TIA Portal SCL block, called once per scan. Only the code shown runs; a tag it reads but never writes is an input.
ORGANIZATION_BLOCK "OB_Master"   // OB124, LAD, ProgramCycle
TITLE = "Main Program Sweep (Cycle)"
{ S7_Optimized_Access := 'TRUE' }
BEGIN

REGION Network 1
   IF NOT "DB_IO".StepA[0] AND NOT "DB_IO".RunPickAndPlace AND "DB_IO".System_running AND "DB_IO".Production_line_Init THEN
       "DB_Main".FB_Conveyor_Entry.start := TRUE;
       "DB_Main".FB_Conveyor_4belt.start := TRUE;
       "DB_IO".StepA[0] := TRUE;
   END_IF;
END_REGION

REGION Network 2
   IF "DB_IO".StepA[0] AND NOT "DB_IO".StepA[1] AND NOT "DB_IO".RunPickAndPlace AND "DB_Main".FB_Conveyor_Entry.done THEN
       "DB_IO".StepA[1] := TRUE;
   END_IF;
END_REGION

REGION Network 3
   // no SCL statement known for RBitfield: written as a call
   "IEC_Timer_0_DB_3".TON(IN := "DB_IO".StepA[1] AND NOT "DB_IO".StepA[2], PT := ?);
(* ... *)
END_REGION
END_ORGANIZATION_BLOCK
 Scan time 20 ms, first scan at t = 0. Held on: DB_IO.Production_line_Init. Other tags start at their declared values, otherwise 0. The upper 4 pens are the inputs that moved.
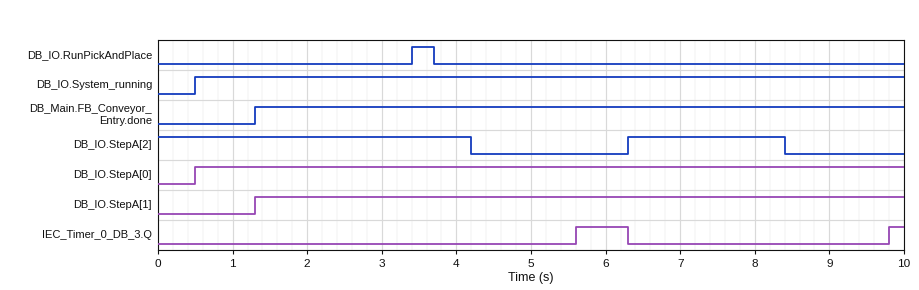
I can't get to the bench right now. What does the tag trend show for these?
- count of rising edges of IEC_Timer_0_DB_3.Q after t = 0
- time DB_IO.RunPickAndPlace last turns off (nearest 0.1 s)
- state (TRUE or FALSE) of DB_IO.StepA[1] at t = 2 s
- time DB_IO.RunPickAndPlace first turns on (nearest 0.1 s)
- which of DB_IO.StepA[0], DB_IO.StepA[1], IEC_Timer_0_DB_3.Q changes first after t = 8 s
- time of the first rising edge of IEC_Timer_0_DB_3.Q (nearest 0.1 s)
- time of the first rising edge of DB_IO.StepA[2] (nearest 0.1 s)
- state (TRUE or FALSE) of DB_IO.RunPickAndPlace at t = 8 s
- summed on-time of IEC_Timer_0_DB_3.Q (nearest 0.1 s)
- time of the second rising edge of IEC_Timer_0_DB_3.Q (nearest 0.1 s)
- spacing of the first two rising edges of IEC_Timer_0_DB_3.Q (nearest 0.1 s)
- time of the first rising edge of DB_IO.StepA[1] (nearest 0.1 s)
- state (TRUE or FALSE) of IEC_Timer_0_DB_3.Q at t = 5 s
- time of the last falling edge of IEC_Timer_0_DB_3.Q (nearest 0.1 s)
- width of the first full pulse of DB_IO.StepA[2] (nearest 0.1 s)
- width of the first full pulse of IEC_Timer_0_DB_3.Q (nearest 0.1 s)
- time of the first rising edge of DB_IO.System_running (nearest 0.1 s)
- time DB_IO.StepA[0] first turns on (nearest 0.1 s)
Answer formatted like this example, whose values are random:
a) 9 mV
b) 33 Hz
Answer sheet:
a) 2
b) 3.7 s
c) TRUE
d) 3.4 s
e) IEC_Timer_0_DB_3.Q
f) 5.6 s
g) 6.3 s
h) FALSE
i) 0.9 s
j) 9.8 s
k) 4.2 s
l) 1.3 s
m) FALSE
n) 6.3 s
o) 2.1 s
p) 0.7 s
q) 0.5 s
r) 0.5 s
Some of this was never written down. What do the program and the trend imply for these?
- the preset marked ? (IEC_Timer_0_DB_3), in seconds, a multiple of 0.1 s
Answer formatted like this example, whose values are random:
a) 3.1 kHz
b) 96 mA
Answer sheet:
a) 1.4 s
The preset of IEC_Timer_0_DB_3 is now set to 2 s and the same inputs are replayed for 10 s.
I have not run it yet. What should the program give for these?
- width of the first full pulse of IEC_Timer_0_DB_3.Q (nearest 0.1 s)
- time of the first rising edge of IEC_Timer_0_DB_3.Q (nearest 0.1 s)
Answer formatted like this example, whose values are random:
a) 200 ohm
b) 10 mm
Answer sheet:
a) 0.1 s
b) 6.2 s
